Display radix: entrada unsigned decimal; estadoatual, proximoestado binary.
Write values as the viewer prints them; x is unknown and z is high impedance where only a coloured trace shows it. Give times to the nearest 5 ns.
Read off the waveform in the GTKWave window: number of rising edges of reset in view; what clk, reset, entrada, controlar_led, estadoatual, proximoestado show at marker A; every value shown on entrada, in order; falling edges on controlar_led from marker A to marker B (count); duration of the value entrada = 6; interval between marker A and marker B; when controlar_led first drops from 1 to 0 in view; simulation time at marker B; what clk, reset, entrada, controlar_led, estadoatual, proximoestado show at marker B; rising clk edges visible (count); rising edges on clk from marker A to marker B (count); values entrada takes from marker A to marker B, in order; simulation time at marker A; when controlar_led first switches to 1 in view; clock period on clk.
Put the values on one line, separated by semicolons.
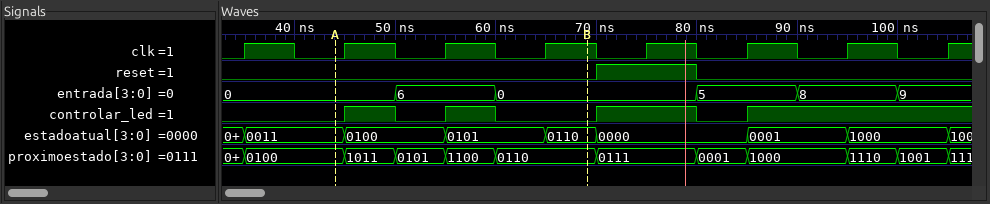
1; clk=0, reset=0, entrada=0, controlar_led=0, estadoatual=0011, proximoestado=0100; 0, 6, 0, 5, 8, 9; 2; 10 ns; 25 ns; 50 ns; 70 ns; clk=1, reset=0, entrada=0, controlar_led=0, estadoatual=0110, proximoestado=0110; 8; 3; 0, 6, 0; 45 ns; 45 ns; 10 ns
